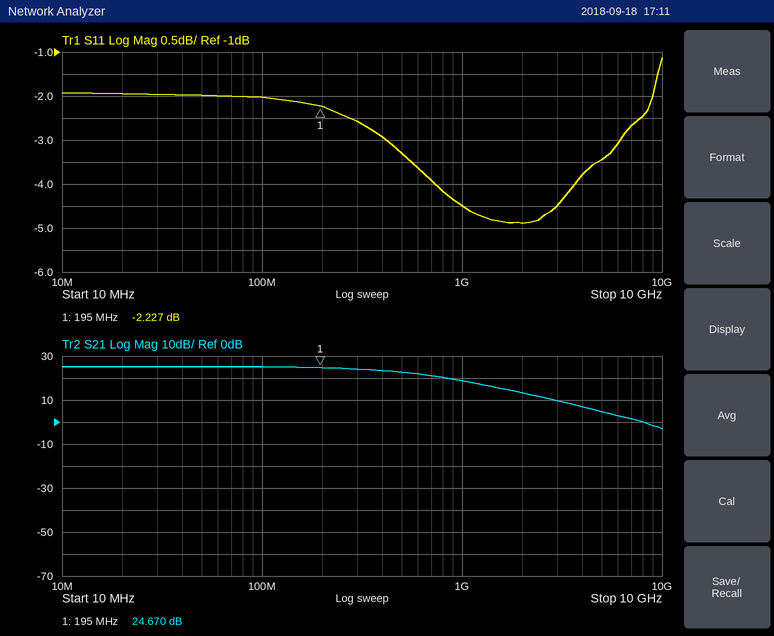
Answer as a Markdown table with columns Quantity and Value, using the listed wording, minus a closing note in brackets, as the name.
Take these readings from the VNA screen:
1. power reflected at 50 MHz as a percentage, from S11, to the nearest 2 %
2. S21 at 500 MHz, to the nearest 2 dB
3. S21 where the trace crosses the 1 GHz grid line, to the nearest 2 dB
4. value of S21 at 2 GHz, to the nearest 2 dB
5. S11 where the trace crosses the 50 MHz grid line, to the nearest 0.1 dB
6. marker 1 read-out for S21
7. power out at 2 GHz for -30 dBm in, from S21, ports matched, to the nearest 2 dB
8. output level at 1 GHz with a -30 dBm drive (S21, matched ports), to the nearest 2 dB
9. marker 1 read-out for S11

| Quantity | Value |
|---|---|
| power reflected at 50 MHz as a percentage, from S11, to the nearest 2 % | 64 % |
| S21 at 500 MHz, to the nearest 2 dB | 22 dB |
| S21 where the trace crosses the 1 GHz grid line, to the nearest 2 dB | 18 dB |
| value of S21 at 2 GHz, to the nearest 2 dB | 14 dB |
| S11 where the trace crosses the 50 MHz grid line, to the nearest 0.1 dB | -2.0 dB |
| marker 1 read-out for S21 | 24.670 dB |
| power out at 2 GHz for -30 dBm in, from S21, ports matched, to the nearest 2 dB | -16 dBm |
| output level at 1 GHz with a -30 dBm drive (S21, matched ports), to the nearest 2 dB | -12 dBm |
| marker 1 read-out for S11 | -2.227 dB |
